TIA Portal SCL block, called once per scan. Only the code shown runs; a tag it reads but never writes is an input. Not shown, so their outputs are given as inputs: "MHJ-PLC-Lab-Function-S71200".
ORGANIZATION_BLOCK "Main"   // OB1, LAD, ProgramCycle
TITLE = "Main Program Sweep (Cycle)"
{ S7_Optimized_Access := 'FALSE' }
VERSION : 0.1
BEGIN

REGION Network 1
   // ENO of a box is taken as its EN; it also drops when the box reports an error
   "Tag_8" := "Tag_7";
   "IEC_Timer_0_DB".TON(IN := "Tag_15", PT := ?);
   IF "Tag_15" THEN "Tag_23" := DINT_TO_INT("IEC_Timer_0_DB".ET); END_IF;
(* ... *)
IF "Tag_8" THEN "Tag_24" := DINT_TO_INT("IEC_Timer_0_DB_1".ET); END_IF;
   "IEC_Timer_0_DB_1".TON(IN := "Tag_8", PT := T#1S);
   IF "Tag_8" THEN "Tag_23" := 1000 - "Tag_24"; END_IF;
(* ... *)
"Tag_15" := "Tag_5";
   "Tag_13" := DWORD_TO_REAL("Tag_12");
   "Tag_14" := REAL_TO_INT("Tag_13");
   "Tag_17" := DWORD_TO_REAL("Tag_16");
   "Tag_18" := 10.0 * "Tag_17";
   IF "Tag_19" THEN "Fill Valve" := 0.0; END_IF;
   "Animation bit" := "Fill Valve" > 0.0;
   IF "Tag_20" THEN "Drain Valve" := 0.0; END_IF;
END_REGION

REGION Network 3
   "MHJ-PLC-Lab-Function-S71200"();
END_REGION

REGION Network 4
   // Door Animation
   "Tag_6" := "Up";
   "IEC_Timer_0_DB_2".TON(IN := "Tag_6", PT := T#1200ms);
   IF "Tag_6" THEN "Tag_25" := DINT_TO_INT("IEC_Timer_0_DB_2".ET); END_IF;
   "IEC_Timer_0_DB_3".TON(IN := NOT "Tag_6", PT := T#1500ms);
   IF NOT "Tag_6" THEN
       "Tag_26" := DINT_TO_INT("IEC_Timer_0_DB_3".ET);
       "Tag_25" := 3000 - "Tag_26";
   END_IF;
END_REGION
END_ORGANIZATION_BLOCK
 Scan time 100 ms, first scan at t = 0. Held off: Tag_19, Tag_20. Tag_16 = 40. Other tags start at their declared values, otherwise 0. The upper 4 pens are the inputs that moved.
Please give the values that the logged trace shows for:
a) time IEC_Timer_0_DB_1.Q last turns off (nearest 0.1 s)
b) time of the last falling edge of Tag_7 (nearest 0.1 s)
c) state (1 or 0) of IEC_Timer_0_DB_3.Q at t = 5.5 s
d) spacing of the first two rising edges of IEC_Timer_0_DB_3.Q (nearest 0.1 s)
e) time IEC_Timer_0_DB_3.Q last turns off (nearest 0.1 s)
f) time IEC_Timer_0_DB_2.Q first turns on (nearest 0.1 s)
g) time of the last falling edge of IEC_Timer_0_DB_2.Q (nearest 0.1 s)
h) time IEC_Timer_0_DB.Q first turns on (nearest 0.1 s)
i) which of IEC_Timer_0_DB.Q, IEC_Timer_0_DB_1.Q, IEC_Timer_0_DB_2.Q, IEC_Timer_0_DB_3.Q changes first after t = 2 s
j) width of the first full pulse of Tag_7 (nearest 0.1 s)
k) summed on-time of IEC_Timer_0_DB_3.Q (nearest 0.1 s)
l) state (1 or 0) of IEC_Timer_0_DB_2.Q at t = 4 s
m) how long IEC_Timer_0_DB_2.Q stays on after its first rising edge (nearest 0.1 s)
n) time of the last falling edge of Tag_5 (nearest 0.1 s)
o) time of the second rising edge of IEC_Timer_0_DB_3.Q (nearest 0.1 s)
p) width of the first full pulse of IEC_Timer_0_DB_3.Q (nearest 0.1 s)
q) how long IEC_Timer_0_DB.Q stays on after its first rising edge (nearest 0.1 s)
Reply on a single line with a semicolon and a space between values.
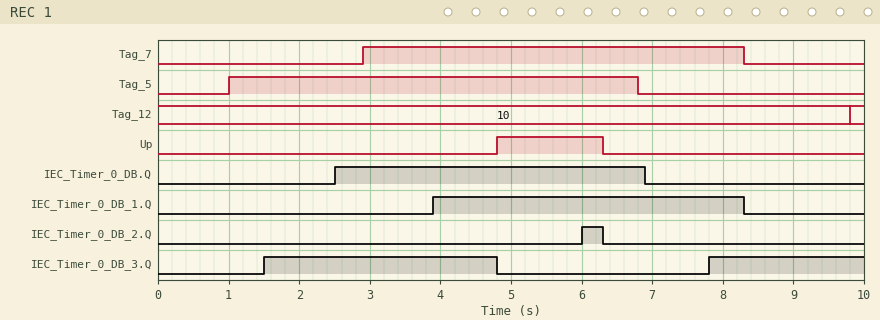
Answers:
8.3 s; 8.3 s; 0; 6.3 s; 4.8 s; 6.0 s; 6.3 s; 2.5 s; IEC_Timer_0_DB.Q; 5.4 s; 5.5 s; 0; 0.3 s; 6.8 s; 7.8 s; 3.3 s; 4.4 s
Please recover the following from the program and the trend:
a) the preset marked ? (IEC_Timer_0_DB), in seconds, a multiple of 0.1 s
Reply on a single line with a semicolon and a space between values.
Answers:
1.4 s
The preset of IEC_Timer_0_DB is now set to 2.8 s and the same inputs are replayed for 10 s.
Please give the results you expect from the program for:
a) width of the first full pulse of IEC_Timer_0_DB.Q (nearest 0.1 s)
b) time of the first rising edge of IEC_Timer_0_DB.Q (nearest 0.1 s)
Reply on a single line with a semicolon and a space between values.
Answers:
3.0 s; 3.9 s
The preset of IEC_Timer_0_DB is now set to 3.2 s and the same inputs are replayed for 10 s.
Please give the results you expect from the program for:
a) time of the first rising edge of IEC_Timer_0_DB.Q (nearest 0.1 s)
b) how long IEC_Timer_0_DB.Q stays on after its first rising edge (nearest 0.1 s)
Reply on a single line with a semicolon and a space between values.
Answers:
4.3 s; 2.6 s
